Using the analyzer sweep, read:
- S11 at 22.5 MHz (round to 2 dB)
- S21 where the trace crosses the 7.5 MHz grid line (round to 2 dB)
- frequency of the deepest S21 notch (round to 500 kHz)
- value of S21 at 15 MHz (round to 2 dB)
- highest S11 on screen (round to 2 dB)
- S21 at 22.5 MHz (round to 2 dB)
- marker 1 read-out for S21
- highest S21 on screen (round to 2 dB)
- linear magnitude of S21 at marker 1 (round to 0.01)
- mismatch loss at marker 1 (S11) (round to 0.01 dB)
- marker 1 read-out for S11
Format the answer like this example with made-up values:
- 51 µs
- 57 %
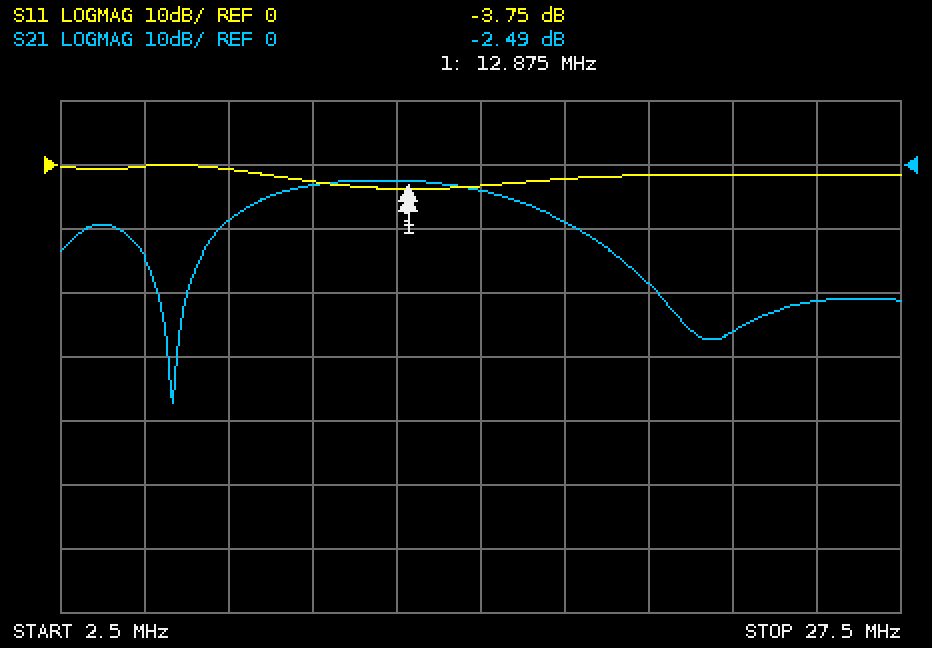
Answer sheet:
- -2 dB
- -8 dB
- 6.0 MHz
- -4 dB
- 0 dB
- -26 dB
- -2.49 dB
- -2 dB
- 0.75
- 2.38 dB
- -3.75 dB
